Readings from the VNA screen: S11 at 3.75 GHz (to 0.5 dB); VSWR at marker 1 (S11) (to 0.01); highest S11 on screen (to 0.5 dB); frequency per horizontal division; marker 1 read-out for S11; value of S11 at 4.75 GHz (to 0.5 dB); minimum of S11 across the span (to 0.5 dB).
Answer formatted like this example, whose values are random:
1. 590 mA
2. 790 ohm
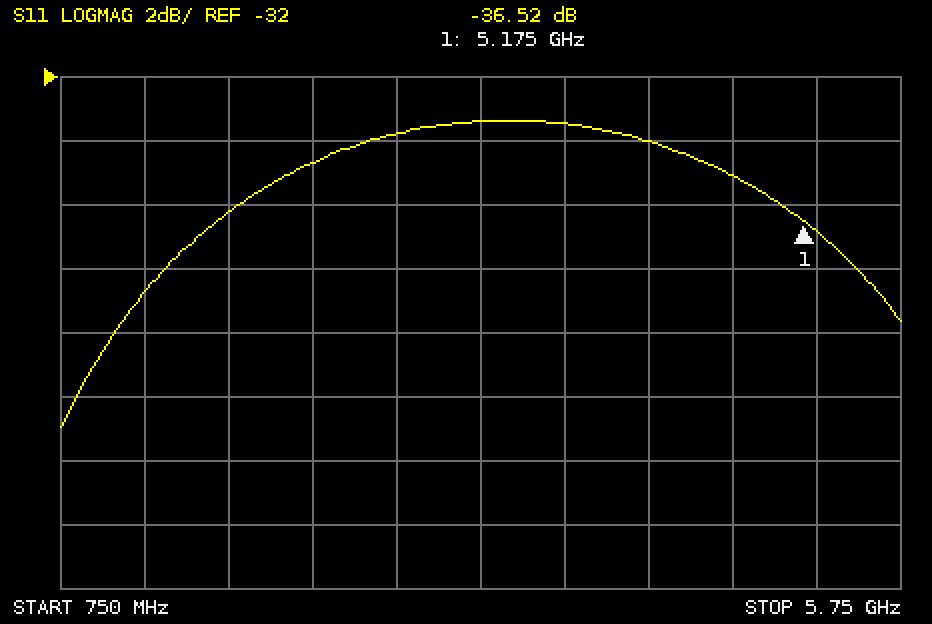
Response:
1. -33.5 dB
2. 1.03
3. -33.5 dB
4. 500 MHz
5. -36.52 dB
6. -35.0 dB
7. -43.0 dB
